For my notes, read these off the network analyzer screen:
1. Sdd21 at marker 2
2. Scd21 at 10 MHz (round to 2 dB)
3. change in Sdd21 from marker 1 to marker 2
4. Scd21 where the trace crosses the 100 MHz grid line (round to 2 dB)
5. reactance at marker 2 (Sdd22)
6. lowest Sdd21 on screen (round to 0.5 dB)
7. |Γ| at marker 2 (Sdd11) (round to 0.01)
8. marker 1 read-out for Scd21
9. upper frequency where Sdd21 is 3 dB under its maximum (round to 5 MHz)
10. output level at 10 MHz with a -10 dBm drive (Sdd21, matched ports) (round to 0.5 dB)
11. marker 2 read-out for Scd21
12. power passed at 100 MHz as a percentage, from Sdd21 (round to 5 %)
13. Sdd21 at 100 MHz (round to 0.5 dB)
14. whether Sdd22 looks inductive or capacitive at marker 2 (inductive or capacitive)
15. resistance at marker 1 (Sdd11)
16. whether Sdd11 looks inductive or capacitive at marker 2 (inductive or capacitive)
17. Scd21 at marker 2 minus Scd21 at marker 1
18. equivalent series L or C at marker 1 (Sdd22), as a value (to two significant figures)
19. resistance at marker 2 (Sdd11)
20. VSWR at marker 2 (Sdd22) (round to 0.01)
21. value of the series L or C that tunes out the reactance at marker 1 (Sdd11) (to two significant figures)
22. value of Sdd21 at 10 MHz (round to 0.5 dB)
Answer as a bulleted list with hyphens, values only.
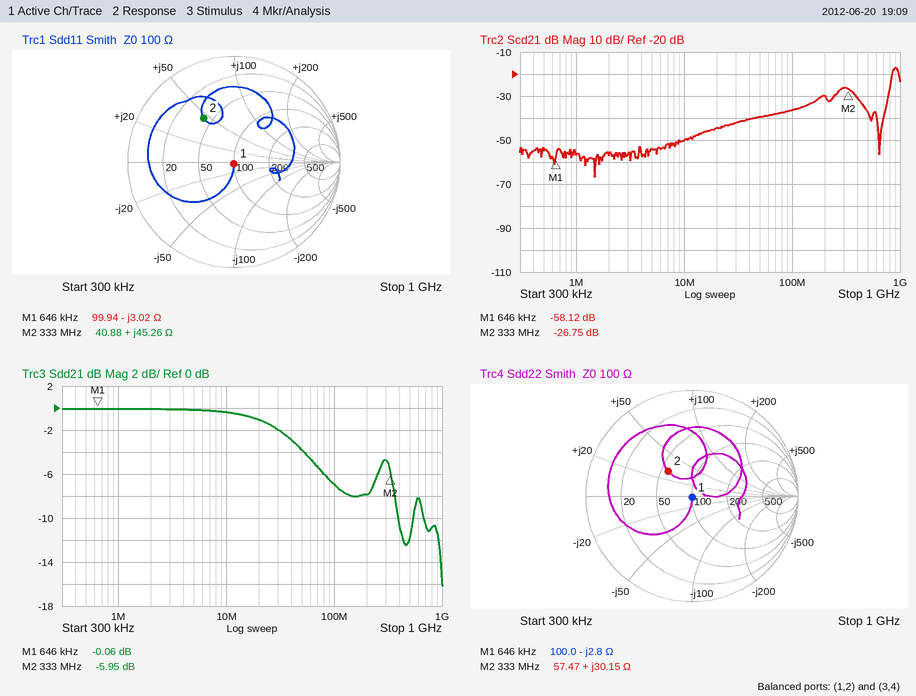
- -5.95 dB
- -50 dB
- -5.89 dB
- -36 dB
- +30.15 Ω
- -16.0 dB
- 0.50
- -58.12 dB
- 40 MHz
- -10.5 dBm
- -26.75 dB
- 20 %
- -7.0 dB
- inductive
- 99.94 Ω
- inductive
- 31.37 dB
- 88 nF
- 40.88 Ω
- 1.96
- 740 nH
- -0.5 dB
